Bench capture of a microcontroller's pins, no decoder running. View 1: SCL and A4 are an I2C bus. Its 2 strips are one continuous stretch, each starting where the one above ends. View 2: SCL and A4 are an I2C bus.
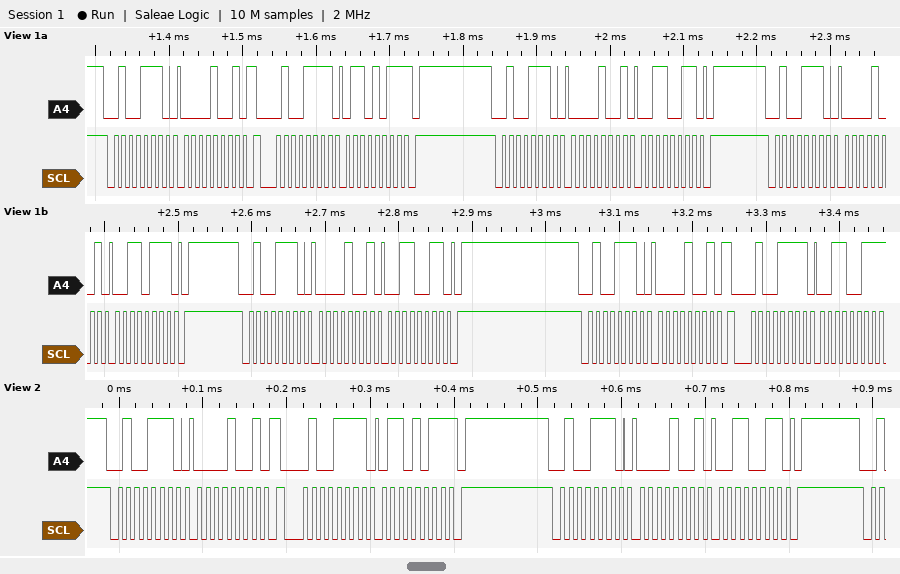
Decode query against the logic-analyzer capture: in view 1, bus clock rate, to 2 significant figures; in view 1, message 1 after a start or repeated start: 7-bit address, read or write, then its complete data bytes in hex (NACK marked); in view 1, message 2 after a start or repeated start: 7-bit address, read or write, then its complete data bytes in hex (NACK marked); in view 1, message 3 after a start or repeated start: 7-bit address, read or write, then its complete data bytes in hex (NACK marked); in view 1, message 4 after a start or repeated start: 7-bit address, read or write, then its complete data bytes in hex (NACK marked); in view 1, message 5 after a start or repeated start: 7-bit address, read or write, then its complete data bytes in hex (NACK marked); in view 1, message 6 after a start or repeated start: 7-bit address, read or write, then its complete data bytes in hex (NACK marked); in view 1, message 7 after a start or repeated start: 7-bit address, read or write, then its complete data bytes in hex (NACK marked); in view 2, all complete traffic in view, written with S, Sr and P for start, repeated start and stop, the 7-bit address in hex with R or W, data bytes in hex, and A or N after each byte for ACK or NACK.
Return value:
100 kHz
0x27 write: 09
0x27 read: 6B NACK
0x27 write: 09 33
0x27 write: 09 37
0x27 write: 09 33
0x27 write: 09
0x27 read: 33 NACK
S 27W A 09 A Sr 27R A 6B N P S 27W A 09 A 33 A P
